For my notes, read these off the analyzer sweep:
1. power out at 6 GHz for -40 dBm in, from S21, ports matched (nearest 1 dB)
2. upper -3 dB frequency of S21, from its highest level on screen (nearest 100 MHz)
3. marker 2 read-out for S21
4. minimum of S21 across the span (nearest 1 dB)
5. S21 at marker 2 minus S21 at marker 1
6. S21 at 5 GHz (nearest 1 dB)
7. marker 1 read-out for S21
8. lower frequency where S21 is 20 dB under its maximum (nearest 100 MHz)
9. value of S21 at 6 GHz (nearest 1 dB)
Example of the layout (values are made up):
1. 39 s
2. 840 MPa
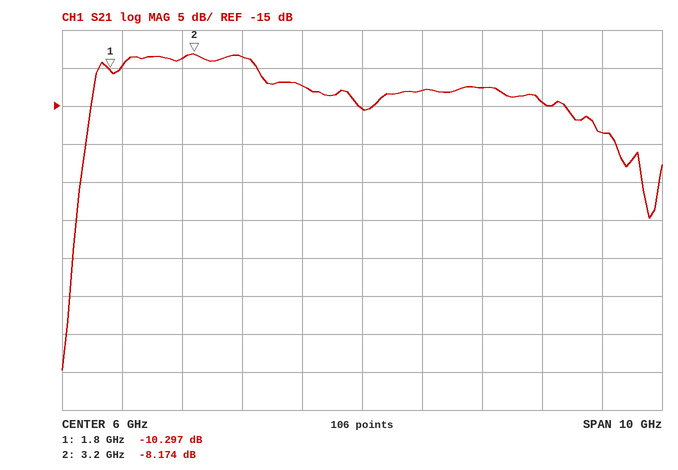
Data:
1. -55 dBm
2. 4.3 GHz
3. -8.174 dB
4. -50 dB
5. 2.123 dB
6. -12 dB
7. -10.297 dB
8. 1.3 GHz
9. -15 dB
